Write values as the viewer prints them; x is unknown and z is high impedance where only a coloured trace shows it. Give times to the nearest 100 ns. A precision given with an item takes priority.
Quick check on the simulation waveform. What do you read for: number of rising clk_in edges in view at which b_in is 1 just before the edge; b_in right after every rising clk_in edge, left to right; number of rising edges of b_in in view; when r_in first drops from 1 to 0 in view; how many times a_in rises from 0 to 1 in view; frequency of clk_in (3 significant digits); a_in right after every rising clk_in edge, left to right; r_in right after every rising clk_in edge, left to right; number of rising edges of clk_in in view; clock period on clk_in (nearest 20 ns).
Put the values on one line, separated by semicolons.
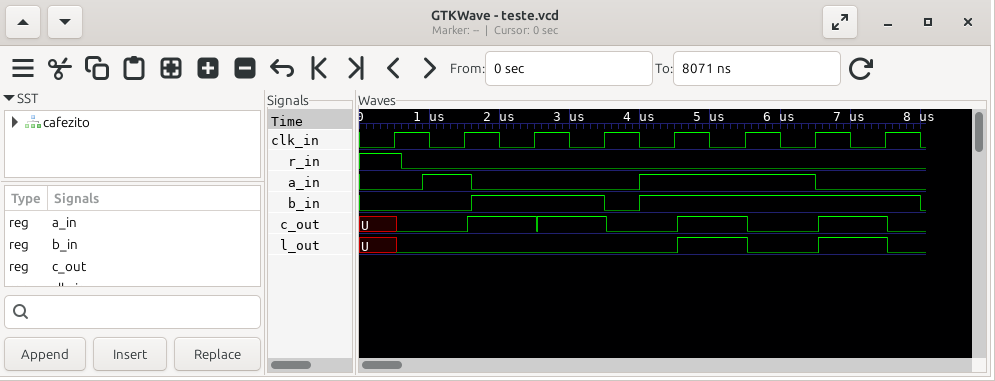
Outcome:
6; 0 0 1 0 1 1 1 1; 2; 600 ns; 2; 1.00 MHz; 0 1 0 0 1 1 0 0; 1 0 0 0 0 0 0 0; 8; 1000 ns
